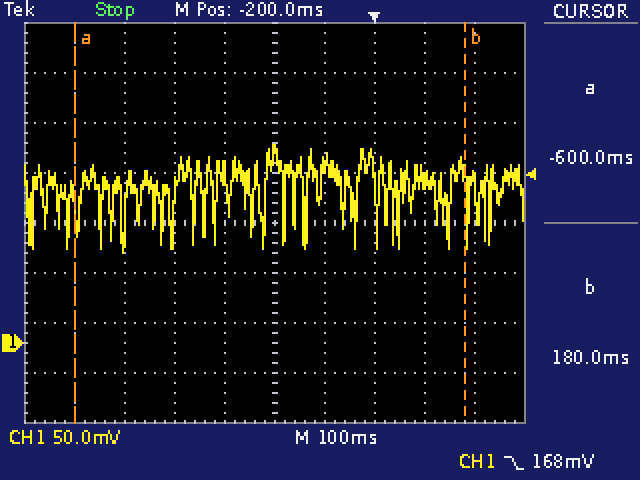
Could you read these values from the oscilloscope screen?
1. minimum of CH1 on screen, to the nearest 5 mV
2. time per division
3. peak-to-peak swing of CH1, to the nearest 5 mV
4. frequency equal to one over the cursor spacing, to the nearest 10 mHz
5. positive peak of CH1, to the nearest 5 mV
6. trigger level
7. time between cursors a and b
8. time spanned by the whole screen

90 mV
100 ms
110 mV
1.28 Hz
200 mV
168 mV
780 ms
1 s
